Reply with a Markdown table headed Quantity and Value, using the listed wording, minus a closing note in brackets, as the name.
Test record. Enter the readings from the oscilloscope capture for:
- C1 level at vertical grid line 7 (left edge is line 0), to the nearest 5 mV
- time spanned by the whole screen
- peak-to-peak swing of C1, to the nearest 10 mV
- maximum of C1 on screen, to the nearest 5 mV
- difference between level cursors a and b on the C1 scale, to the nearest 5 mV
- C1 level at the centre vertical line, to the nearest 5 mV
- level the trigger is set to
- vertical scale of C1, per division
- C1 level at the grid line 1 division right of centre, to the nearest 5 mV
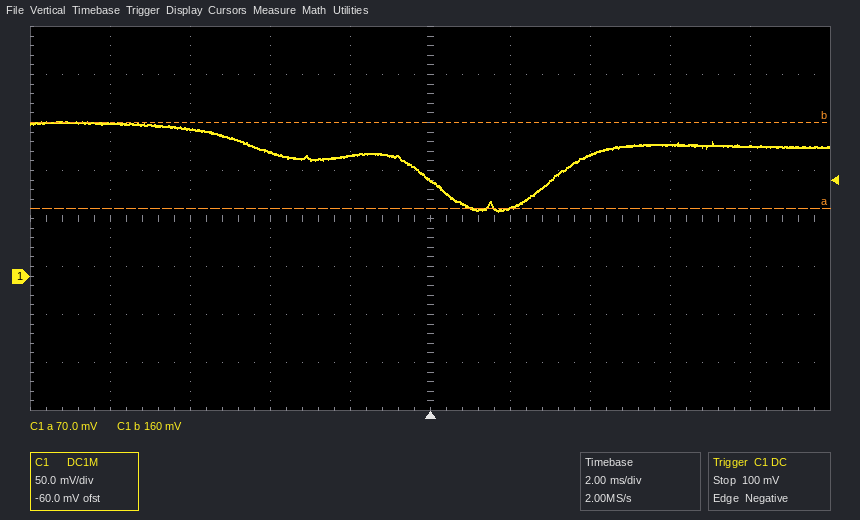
| Quantity | Value |
|---|---|
| C1 level at vertical grid line 7 (left edge is line 0), to the nearest 5 mV | 125 mV |
| time spanned by the whole screen | 20 ms |
| peak-to-peak swing of C1, to the nearest 10 mV | 90 mV |
| maximum of C1 on screen, to the nearest 5 mV | 160 mV |
| difference between level cursors a and b on the C1 scale, to the nearest 5 mV | 90 mV |
| C1 level at the centre vertical line, to the nearest 5 mV | 100 mV |
| level the trigger is set to | 100 mV |
| vertical scale of C1, per division | 50 mV |
| C1 level at the grid line 1 division right of centre, to the nearest 5 mV | 70 mV |
